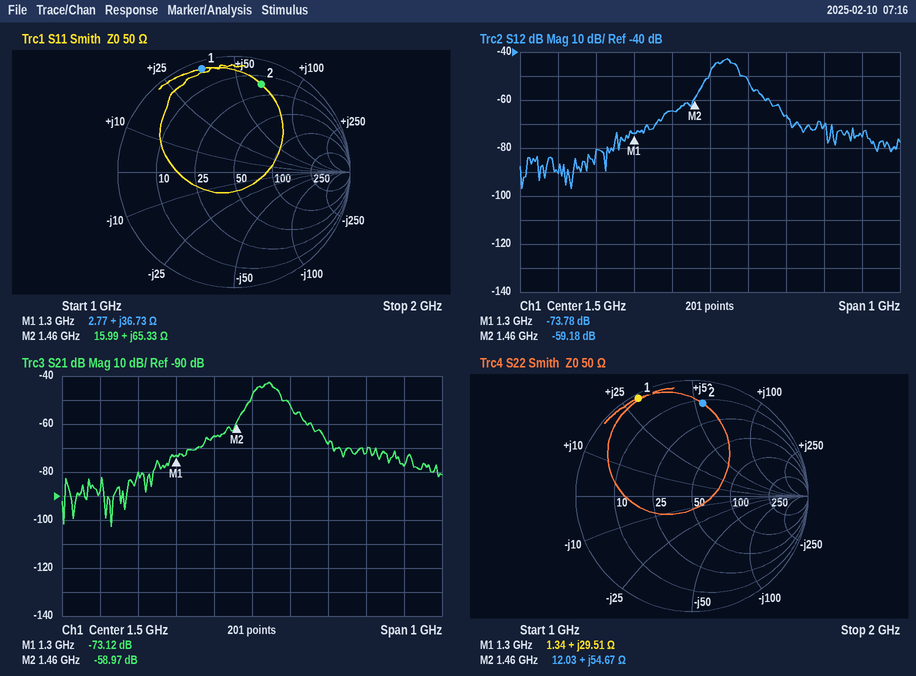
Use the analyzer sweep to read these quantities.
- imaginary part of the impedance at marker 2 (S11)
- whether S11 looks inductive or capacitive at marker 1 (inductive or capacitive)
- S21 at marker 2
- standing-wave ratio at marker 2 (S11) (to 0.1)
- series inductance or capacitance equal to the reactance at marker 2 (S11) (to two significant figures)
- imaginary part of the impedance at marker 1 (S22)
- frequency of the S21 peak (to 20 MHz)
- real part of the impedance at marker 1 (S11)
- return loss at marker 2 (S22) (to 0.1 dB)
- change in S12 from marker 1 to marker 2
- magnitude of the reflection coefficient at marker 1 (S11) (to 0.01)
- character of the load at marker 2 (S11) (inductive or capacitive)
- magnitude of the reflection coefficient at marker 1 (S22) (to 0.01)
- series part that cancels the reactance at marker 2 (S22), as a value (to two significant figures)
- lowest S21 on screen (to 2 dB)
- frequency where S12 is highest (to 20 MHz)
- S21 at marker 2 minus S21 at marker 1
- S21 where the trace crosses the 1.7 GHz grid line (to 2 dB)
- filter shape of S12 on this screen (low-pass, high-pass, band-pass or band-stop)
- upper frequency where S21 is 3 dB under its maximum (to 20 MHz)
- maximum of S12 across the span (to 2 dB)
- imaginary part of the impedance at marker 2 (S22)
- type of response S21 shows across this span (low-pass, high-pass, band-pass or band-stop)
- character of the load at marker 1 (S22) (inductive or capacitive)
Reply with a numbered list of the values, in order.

1. +65.33 Ω
2. inductive
3. -58.97 dB
4. 8.7
5. 7.1 nH
6. +29.51 Ω
7. 1.54 GHz
8. 2.77 Ω
9. 1.9 dB
10. 14.60 dB
11. 0.93
12. inductive
13. 0.96
14. 2.0 pF
15. -102 dB
16. 1.54 GHz
17. 14.15 dB
18. -68 dB
19. band-pass
20. 1.56 GHz
21. -42 dB
22. +54.67 Ω
23. band-pass
24. inductive
